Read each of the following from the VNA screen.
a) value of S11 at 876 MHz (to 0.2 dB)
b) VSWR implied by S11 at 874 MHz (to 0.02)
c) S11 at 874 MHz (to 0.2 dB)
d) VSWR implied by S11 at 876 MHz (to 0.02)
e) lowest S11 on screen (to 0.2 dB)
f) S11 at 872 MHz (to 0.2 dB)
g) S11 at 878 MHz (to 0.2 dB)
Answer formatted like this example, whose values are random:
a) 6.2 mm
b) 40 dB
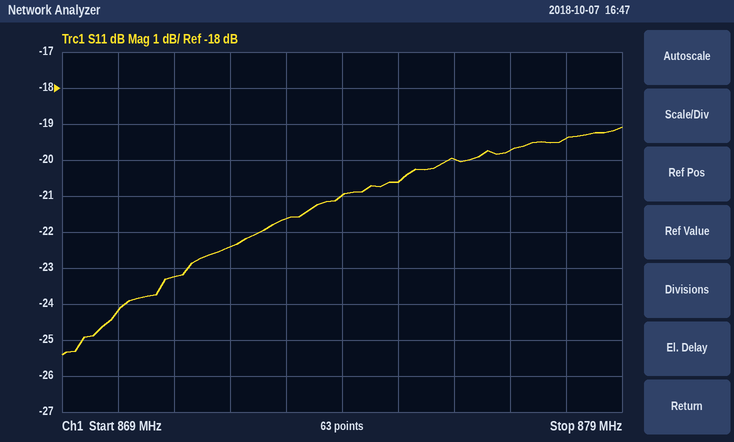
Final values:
a) -20.0 dB
b) 1.20
c) -21.0 dB
d) 1.22
e) -25.4 dB
f) -22.4 dB
g) -19.4 dB
